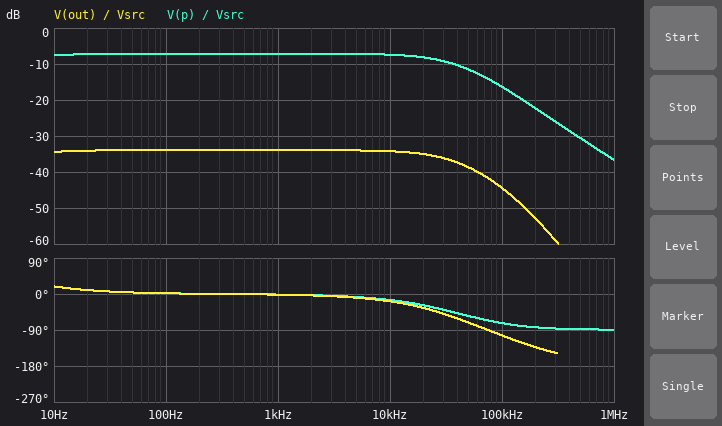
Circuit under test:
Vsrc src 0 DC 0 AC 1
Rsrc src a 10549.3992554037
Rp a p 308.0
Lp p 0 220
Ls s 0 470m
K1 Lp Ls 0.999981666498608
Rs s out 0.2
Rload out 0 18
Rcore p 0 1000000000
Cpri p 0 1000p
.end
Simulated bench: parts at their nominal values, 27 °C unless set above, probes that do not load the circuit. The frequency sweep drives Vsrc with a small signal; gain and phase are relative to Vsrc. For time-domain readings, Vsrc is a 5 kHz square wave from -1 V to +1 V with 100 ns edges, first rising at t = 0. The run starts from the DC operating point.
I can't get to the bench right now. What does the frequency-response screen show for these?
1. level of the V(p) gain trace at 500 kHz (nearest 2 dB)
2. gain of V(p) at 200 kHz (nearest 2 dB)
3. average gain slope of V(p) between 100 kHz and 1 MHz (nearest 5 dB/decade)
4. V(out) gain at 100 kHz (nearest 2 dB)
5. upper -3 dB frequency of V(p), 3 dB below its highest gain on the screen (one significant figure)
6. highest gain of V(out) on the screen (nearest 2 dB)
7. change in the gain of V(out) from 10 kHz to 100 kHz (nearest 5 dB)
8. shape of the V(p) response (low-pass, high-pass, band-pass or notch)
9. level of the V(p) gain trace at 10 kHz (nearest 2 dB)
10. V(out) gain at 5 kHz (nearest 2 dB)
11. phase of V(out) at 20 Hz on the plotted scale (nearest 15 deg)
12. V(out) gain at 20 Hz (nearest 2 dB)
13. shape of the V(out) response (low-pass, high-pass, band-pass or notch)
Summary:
-30 dB
-22 dB
-20 dB/decade
-44 dB
40 kHz
-34 dB
-10 dB
low-pass
-8 dB
-34 dB
15 deg
-34 dB
low-pass
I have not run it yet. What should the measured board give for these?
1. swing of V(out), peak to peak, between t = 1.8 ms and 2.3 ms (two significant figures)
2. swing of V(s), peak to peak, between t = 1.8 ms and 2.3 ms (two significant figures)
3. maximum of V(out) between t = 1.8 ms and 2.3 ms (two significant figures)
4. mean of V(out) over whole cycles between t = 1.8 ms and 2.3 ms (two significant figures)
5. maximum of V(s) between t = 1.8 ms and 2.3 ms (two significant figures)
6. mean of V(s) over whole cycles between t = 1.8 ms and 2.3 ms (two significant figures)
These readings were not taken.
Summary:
40 mV
41 mV
39 mV
19 mV
40 mV
19 mV
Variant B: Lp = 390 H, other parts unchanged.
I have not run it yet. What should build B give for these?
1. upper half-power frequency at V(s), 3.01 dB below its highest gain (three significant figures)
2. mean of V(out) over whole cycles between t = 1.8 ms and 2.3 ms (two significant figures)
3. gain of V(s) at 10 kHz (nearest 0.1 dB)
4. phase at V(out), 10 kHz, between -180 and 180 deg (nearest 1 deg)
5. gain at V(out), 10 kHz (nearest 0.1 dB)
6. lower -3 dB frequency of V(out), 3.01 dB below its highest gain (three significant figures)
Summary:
26.5 kHz
19 mV
-34.5 dB
-24 deg
-34.6 dB
2.58 Hz
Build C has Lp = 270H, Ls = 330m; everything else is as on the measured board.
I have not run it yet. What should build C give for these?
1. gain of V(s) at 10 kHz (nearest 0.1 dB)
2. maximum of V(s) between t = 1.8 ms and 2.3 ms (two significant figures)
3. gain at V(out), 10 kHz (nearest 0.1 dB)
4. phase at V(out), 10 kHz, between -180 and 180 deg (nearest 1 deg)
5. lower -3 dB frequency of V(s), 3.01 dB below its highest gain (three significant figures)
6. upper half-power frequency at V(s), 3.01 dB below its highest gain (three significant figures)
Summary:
-34.5 dB
40 mV
-34.6 dB
-23 deg
3.70 Hz
26.3 kHz
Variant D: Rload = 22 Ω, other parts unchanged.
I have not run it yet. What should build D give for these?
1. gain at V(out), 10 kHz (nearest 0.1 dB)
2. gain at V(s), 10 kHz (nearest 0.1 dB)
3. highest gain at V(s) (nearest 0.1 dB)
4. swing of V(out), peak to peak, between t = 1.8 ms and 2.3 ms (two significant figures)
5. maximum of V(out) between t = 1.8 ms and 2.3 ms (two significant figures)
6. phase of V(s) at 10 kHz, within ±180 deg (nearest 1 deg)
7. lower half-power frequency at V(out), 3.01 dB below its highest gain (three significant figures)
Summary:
-33.4 dB
-33.3 dB
-32.9 dB
45 mV
44 mV
-20 deg
3.84 Hz
